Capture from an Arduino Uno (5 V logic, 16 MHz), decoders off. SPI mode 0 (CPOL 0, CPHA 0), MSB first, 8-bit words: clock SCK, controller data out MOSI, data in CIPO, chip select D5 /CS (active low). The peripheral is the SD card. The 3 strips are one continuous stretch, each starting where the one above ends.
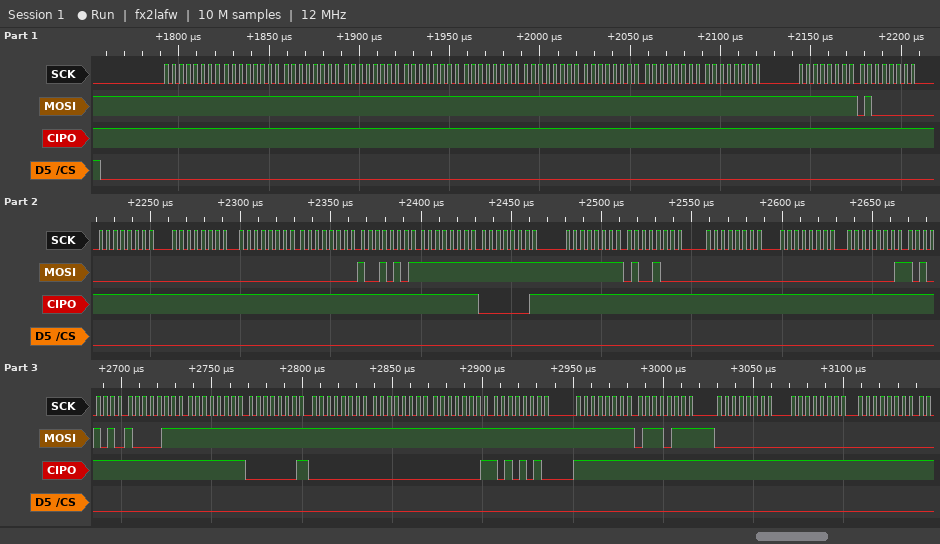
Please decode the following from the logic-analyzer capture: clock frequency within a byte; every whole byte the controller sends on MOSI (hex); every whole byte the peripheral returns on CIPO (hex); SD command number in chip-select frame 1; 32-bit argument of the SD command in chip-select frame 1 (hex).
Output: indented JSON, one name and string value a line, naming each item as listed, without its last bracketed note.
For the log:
{
  "clock frequency within a byte": "250 kHz",
  "every whole byte the controller sends on MOSI": "0xFF 0xFF 0xFF 0xFF 0xFF 0xFF 0xFF 0xFF 0xFF 0xFF 0xFF 0x40 0x00 0x00 0x00 0x00 0x95 0xFF 0xFF 0xFF 0x48 0x00 0x00 0x01 0xAA 0x87 0xFF 0xFF 0xFF 0xFF 0xFF 0xFF 0xFF 0x77 0x00 0x00 0x00",
  "every whole byte the peripheral returns on CIPO": "0xFF 0xFF 0xFF 0xFF 0xFF 0xFF 0xFF 0xFF 0xFF 0xFF 0xFF 0xFF 0xFF 0xFF 0xFF 0xFF 0xFF 0xFF 0x01 0xFF 0xFF 0xFF 0xFF 0xFF 0xFF 0xFF 0xFF 0x01 0x00 0x00 0x01 0xAA 0xFF 0xFF 0xFF 0xFF 0xFF",
  "SD command number in chip-select frame 1": "CMD0",
  "32-bit argument of the SD command in chip-select frame 1": "0x00000000"
}
